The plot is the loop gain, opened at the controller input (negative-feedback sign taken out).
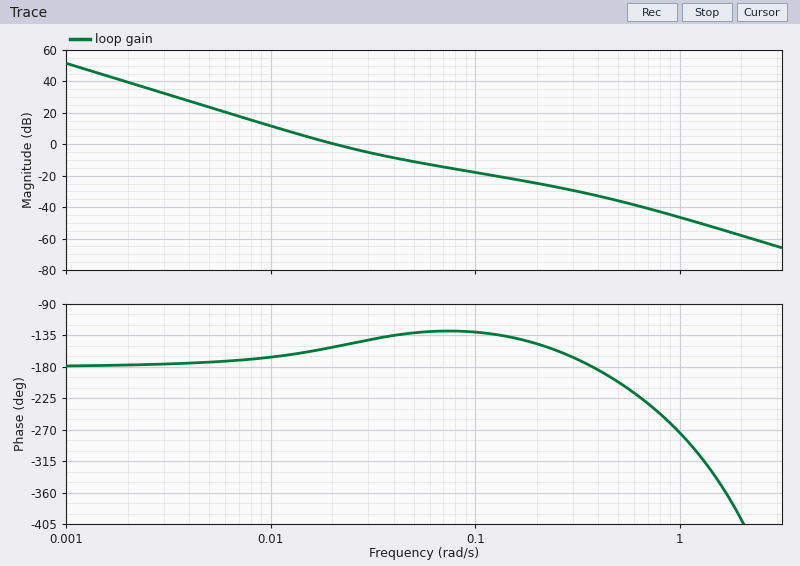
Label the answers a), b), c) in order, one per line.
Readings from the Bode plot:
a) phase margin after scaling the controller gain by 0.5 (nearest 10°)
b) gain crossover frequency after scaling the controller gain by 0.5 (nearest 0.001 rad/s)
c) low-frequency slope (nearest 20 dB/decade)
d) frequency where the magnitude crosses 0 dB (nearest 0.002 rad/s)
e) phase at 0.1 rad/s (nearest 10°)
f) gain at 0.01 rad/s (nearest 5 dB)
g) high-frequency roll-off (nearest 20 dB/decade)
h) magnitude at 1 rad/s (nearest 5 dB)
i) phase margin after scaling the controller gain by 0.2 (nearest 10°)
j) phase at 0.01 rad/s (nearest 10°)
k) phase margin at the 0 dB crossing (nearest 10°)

a) 20°
b) 0.014 rad/s
c) -40 dB/decade
d) 0.020 rad/s
e) -130°
f) 10 dB
g) -40 dB/decade
h) -45 dB
i) 10°
j) -170°
k) 30°
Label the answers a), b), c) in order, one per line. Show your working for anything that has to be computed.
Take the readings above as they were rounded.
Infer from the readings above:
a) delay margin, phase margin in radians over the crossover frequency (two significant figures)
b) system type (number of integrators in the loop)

a) 30 × π / 180 / 0.02 = 26 s
b) 2
